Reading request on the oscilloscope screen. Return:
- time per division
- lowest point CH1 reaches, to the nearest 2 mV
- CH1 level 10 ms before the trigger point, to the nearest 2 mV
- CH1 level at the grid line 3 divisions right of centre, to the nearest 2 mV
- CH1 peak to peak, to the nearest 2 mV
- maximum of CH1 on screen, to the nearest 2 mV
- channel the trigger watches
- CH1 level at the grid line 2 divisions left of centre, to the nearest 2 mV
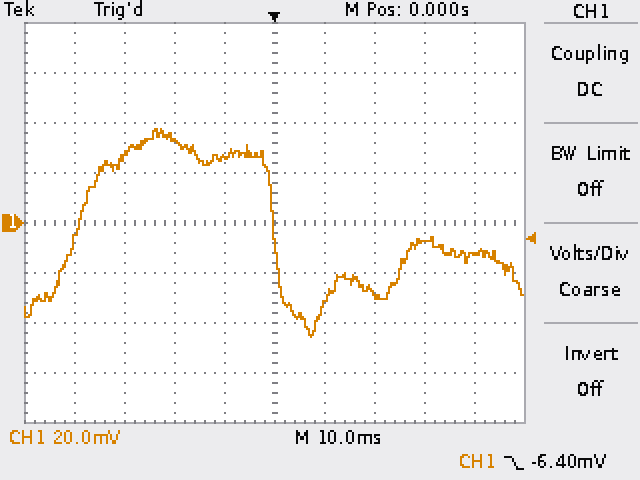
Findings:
10 ms
-46 mV
26 mV
-8 mV
84 mV
38 mV
CH1
34 mV
